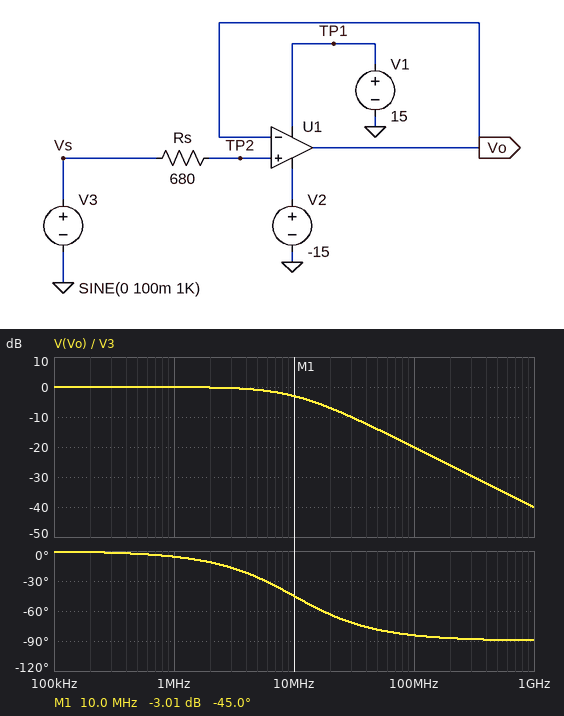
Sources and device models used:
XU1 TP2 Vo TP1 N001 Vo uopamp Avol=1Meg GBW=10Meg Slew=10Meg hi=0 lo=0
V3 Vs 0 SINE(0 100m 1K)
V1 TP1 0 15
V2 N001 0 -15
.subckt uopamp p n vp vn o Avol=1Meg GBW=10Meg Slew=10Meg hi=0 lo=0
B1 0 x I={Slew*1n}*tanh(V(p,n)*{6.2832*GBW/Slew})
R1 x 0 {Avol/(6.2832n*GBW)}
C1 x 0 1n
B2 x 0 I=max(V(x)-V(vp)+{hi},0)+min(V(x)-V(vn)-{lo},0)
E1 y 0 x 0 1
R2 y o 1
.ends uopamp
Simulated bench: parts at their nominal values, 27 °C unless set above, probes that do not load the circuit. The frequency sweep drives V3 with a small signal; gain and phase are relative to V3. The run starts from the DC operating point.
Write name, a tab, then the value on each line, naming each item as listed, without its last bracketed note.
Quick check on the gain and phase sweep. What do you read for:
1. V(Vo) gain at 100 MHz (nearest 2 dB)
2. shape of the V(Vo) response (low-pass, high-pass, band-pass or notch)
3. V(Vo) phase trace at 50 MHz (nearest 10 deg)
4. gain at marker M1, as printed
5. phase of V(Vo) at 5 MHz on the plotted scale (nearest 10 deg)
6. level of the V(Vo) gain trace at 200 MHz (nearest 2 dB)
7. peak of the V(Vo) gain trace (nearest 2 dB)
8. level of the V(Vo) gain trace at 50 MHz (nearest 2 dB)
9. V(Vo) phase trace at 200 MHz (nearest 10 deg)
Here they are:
V(Vo) gain at 100 MHz	-20 dB
shape of the V(Vo) response	low-pass
V(Vo) phase trace at 50 MHz	-80 deg
gain at marker M1, as printed	-3.01 dB
phase of V(Vo) at 5 MHz on the plotted scale	-30 deg
level of the V(Vo) gain trace at 200 MHz	-26 dB
peak of the V(Vo) gain trace	0 dB
level of the V(Vo) gain trace at 50 MHz	-14 dB
V(Vo) phase trace at 200 MHz	-90 deg
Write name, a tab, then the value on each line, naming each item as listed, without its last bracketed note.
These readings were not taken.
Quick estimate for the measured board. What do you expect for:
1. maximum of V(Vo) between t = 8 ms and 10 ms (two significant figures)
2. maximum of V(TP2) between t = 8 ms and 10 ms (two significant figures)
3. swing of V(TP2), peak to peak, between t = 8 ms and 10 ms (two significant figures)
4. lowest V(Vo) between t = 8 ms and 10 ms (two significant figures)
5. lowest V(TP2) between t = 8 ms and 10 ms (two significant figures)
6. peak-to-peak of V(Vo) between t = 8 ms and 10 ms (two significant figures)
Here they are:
maximum of V(Vo) between t = 8 ms and 10 ms	100 mV
maximum of V(TP2) between t = 8 ms and 10 ms	100 mV
swing of V(TP2), peak to peak, between t = 8 ms and 10 ms	200 mV
lowest V(Vo) between t = 8 ms and 10 ms	-100 mV
lowest V(TP2) between t = 8 ms and 10 ms	-100 mV
peak-to-peak of V(Vo) between t = 8 ms and 10 ms	200 mV
